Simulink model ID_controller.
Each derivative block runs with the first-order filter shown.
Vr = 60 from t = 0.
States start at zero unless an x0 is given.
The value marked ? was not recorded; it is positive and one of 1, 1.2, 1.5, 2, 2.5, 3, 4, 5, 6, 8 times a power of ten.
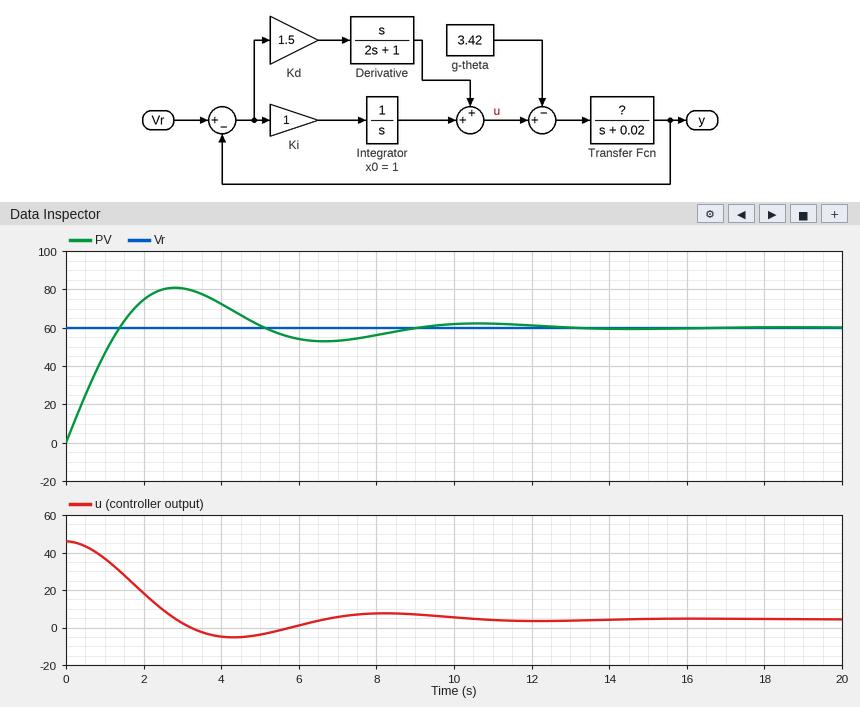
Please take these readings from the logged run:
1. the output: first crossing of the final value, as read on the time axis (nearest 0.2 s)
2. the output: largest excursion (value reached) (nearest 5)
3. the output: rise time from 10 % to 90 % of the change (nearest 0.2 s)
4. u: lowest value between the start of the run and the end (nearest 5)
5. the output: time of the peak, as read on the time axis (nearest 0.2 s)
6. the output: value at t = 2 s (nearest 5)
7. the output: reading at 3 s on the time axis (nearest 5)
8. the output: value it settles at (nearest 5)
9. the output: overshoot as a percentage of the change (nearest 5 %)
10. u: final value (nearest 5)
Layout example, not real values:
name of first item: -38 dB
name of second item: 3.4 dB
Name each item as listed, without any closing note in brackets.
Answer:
the output: first crossing of the final value, as read on the time axis: 1.4 s
the output: largest excursion (value reached): 80
the output: rise time from 10 % to 90 % of the change: 1.0 s
u: lowest value between the start of the run and the end: -5
the output: time of the peak, as read on the time axis: 2.8 s
the output: value at t = 2 s: 75
the output: reading at 3 s on the time axis: 80
the output: value it settles at: 60
the output: overshoot as a percentage of the change: 35 %
u: final value: 5
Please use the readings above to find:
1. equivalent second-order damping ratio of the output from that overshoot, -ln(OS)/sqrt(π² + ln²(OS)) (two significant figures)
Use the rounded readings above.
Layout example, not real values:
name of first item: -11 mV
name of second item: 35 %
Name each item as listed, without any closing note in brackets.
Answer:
equivalent second-order damping ratio of the output from that overshoot, -ln(OS)/sqrt(π² + ln²(OS)): 0.32
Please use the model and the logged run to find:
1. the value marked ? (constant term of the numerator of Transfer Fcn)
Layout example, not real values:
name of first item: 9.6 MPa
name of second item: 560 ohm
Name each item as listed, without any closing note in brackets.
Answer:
the value marked ?: 1.2
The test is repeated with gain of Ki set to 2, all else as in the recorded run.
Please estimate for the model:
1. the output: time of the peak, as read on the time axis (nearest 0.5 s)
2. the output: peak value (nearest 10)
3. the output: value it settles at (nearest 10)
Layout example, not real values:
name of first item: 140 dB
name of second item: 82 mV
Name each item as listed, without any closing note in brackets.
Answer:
the output: time of the peak, as read on the time axis: 2.0 s
the output: peak value: 90
the output: value it settles at: 60
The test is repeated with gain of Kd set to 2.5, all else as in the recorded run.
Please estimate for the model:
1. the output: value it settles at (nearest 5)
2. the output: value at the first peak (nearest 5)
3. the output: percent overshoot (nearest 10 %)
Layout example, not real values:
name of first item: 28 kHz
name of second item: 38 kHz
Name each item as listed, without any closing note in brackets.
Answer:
the output: value it settles at: 60
the output: value at the first peak: 70
the output: percent overshoot: 20 %
